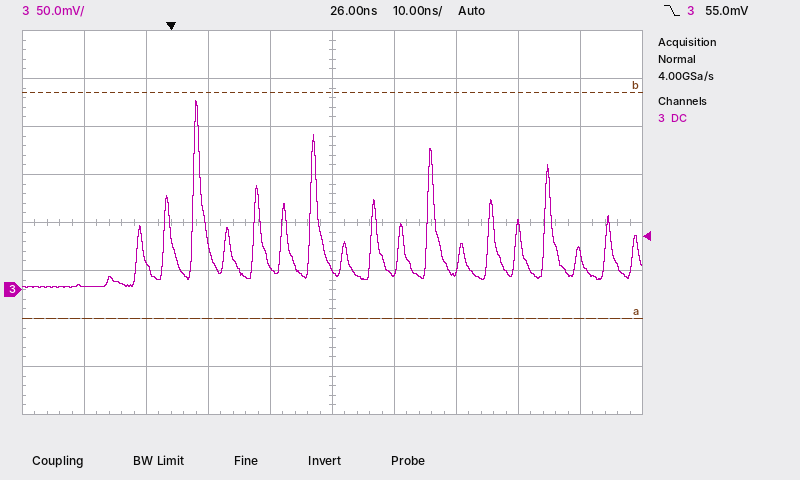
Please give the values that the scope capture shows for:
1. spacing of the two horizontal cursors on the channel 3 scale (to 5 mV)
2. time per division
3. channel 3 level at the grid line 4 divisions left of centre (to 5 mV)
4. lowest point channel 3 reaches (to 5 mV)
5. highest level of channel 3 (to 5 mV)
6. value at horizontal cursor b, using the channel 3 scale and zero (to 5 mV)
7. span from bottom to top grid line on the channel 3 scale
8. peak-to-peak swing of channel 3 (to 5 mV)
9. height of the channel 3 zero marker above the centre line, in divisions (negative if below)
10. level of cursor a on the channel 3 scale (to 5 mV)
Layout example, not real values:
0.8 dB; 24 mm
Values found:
235 mV; 10 ns; 5 mV; 0 mV; 195 mV; 205 mV; 400 mV; 195 mV; -1.4 div; -30 mV
